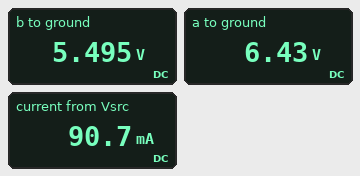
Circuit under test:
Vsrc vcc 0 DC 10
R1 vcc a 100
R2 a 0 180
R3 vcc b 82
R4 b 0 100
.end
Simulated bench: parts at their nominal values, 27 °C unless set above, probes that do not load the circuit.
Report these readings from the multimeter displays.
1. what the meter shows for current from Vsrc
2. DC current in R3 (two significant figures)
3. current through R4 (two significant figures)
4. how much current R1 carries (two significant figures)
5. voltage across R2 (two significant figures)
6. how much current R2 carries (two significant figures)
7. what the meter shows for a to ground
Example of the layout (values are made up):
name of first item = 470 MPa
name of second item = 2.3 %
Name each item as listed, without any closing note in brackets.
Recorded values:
what the meter shows for current from Vsrc = 90.7 mA
DC current in R3 = 55 mA
current through R4 = 55 mA
how much current R1 carries = 36 mA
voltage across R2 = 6.4 V
how much current R2 carries = 36 mA
what the meter shows for a to ground = 6.43 V
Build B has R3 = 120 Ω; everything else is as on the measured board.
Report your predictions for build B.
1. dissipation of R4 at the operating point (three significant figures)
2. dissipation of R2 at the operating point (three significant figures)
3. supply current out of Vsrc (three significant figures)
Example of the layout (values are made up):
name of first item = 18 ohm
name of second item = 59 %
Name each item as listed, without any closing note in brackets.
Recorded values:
dissipation of R4 at the operating point = 207 mW
dissipation of R2 at the operating point = 230 mW
supply current out of Vsrc = 81.2 mA
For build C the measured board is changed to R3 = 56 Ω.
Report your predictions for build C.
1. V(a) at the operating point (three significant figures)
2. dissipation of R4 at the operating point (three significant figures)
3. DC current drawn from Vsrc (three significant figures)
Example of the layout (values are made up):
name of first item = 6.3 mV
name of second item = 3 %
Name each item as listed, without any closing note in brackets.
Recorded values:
V(a) at the operating point = 6.43 V
dissipation of R4 at the operating point = 411 mW
DC current drawn from Vsrc = 99.8 mA
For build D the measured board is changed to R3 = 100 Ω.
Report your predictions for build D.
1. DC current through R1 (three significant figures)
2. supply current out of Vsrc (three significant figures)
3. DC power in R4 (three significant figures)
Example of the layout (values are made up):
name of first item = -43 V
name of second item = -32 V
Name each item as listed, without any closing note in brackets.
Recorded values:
DC current through R1 = 35.7 mA
supply current out of Vsrc = 85.7 mA
DC power in R4 = 250 mW
